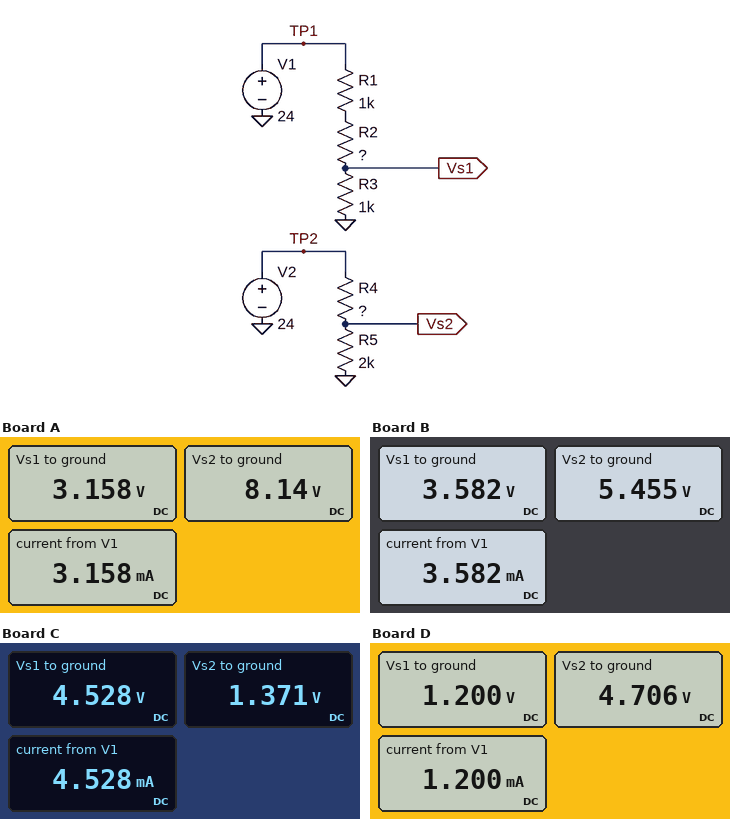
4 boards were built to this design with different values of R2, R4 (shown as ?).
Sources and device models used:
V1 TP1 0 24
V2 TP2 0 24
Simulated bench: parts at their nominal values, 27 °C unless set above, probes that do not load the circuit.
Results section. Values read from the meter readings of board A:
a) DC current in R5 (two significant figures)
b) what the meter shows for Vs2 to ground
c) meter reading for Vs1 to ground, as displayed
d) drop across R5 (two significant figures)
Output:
4.1 mA
8.14 V
3.158 V
8.1 V
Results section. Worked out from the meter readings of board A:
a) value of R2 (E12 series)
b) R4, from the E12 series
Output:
5.6 kΩ
3.9 kΩ
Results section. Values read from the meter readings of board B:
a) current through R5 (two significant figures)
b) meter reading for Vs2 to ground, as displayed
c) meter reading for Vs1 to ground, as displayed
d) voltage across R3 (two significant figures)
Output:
2.7 mA
5.455 V
3.582 V
3.6 V
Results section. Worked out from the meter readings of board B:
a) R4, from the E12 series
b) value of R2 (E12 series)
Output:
6.8 kΩ
4.7 kΩ
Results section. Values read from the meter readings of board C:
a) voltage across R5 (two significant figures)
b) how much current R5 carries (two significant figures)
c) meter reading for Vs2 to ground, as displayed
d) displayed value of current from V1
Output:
1.4 V
690 µA
1.371 V
4.528 mA
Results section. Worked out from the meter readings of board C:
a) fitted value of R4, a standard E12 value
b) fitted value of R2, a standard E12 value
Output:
33 kΩ
3.3 kΩ
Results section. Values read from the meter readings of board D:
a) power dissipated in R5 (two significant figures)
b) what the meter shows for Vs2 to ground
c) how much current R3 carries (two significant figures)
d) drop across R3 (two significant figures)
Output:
11 mW
4.706 V
1.2 mA
1.2 V
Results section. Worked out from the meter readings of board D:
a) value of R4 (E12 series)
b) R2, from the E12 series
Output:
8.2 kΩ
18 kΩ
